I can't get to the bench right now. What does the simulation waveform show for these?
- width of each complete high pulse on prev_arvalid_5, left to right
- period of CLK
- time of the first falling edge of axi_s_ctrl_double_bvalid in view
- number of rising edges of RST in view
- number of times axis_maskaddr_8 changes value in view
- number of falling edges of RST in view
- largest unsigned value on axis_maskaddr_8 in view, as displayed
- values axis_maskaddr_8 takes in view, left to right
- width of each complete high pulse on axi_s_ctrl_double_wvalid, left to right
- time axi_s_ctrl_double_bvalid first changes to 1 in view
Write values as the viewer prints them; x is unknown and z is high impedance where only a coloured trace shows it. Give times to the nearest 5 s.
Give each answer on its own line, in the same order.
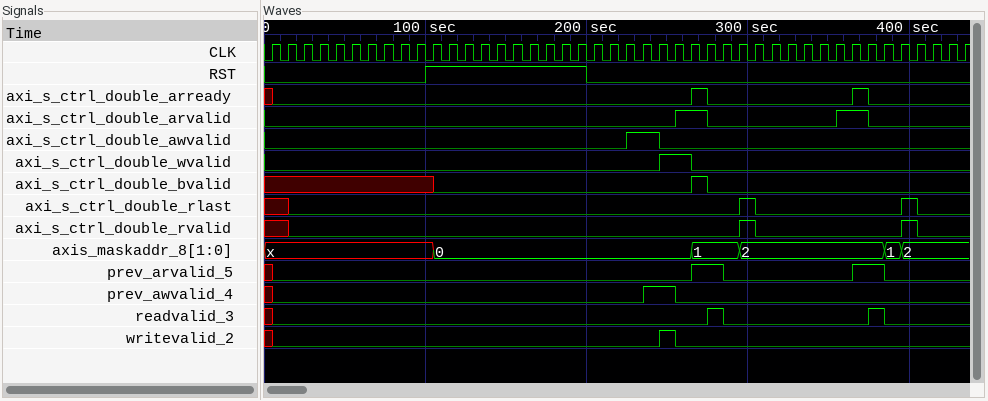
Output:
20 s, 20 s
10 s
275 s
1
5
1
2
x, 0, 1, 2, 1, 2
20 s
265 s
